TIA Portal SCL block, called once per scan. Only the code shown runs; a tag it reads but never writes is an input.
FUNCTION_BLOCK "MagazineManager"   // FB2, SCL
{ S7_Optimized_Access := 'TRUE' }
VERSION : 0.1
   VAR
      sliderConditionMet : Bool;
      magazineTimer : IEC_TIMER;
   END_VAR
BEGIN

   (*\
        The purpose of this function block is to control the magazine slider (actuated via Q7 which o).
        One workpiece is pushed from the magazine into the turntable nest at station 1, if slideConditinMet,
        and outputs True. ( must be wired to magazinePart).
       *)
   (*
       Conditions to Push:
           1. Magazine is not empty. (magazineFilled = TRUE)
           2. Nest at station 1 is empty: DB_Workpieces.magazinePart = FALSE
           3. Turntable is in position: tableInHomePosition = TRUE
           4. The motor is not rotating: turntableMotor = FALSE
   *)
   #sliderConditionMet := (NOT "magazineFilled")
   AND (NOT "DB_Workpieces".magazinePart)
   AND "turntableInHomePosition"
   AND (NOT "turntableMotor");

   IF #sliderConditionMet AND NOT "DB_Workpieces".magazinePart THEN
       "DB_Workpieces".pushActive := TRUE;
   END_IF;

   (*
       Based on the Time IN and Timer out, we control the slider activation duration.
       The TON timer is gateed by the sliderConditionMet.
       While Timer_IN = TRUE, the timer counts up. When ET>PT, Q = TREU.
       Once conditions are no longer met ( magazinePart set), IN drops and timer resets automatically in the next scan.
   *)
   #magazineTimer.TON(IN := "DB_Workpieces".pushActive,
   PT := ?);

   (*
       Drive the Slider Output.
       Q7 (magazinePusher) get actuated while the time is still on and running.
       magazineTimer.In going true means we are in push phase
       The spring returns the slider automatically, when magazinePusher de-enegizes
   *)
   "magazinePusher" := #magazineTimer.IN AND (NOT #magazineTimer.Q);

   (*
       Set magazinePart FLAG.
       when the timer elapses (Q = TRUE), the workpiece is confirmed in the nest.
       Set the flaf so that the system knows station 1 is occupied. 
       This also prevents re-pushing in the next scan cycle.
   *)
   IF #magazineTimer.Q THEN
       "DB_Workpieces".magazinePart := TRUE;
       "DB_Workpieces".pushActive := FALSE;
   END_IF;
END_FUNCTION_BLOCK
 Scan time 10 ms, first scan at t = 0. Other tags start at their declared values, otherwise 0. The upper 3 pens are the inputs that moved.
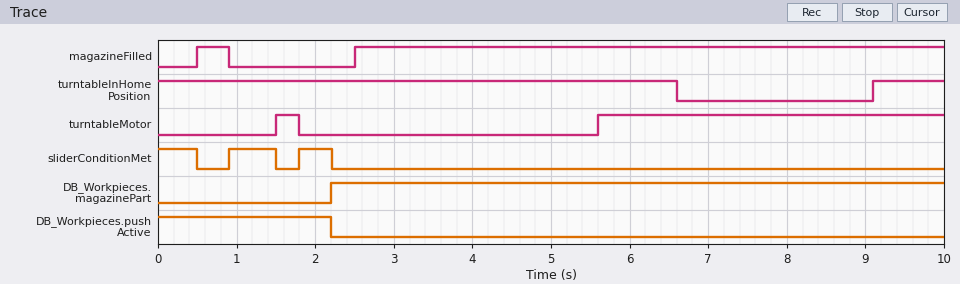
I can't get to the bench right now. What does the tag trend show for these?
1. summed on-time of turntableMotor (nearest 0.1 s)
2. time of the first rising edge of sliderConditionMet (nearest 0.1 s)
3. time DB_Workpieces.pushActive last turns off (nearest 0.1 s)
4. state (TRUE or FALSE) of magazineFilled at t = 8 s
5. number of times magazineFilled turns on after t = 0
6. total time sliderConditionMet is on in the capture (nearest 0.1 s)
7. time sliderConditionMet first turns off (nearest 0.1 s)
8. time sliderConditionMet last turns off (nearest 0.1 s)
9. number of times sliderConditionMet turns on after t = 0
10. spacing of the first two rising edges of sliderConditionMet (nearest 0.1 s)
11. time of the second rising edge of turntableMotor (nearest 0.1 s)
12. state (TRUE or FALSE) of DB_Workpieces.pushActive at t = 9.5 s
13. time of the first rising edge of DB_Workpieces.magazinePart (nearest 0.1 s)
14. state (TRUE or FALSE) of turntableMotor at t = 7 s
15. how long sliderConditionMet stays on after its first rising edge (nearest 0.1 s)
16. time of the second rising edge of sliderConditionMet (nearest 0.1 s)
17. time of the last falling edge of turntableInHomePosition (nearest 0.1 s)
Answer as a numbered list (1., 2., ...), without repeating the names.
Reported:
1. 4.7 s
2. 0.9 s
3. 2.2 s
4. TRUE
5. 2
6. 1.5 s
7. 0.5 s
8. 2.2 s
9. 2
10. 0.9 s
11. 5.6 s
12. FALSE
13. 2.2 s
14. TRUE
15. 0.6 s
16. 1.8 s
17. 6.6 s
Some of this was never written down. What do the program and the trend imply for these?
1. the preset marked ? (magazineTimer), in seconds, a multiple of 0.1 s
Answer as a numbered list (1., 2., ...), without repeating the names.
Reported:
1. 2.2 s
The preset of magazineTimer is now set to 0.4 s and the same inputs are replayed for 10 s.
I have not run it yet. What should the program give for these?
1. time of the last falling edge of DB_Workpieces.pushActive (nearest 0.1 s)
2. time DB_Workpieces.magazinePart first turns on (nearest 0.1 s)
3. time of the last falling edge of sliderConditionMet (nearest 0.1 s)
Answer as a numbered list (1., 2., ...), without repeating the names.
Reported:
1. 0.4 s
2. 0.4 s
3. 0.4 s
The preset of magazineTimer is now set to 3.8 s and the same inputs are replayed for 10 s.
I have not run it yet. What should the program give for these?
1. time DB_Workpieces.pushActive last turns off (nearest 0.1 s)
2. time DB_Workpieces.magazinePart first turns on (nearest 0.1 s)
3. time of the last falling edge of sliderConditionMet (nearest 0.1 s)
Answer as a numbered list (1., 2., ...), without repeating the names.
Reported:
1. 3.8 s
2. 3.8 s
3. 2.5 s
